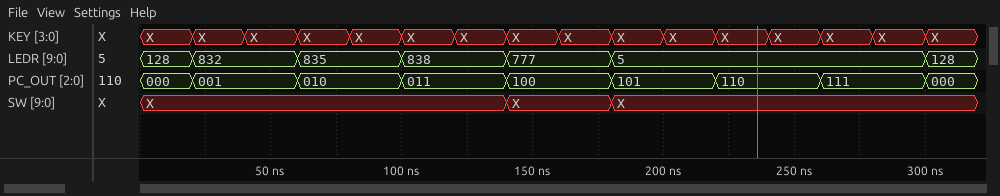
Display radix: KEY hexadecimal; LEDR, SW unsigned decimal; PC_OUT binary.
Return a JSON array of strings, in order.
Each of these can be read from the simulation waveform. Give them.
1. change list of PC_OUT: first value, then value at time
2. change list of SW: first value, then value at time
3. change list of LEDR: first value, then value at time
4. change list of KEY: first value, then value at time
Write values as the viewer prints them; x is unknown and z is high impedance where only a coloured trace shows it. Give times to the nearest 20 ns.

["000, 001 at 20 ns, 010 at 60 ns, 011 at 100 ns, 100 at 140 ns, 101 at 180 ns, 110 at 220 ns, 111 at 260 ns, 000 at 300 ns", "X, X at 140 ns, X at 180 ns", "128, 832 at 20 ns, 835 at 60 ns, 838 at 100 ns, 777 at 140 ns, 5 at 180 ns, 128 at 300 ns", "X, X at 20 ns, X at 40 ns, X at 60 ns, X at 80 ns, X at 100 ns, X at 120 ns, X at 140 ns, X at 160 ns, X at 180 ns, X at 200 ns, X at 220 ns, X at 240 ns, X at 260 ns, X at 280 ns, X at 300 ns"]
